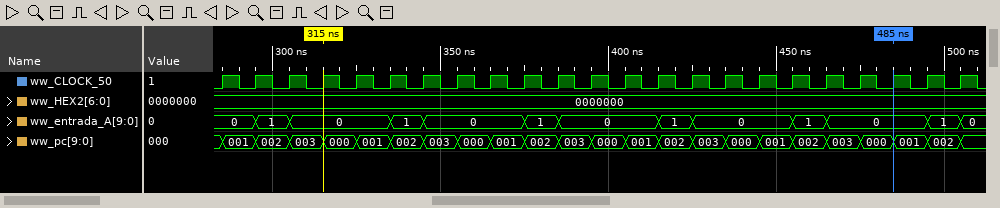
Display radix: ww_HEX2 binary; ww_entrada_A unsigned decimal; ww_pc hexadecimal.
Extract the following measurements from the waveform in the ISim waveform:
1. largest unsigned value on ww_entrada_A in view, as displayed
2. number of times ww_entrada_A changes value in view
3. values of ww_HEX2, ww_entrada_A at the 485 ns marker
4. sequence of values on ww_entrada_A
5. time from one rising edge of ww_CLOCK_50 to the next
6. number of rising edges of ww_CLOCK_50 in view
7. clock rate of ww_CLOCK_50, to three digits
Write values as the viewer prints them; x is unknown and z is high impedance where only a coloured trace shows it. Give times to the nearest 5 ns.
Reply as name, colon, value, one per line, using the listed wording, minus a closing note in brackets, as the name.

largest unsigned value on ww_entrada_A in view, as displayed: 1
number of times ww_entrada_A changes value in view: 12
values of ww_HEX2, ww_entrada_A at the 485 ns marker: ww_HEX2=0000000, ww_entrada_A=0
sequence of values on ww_entrada_A: 0, 1, 0, 1, 0, 1, 0, 1, 0, 1, 0, 1, 0
time from one rising edge of ww_CLOCK_50 to the next: 10 ns
number of rising edges of ww_CLOCK_50 in view: 23
clock rate of ww_CLOCK_50, to three digits: 100 MHz
